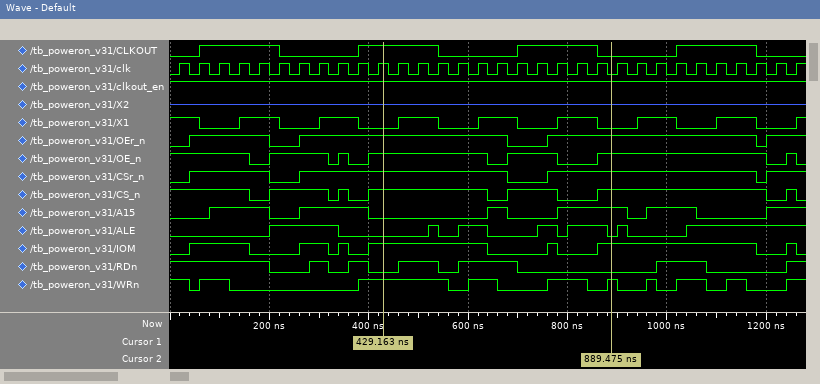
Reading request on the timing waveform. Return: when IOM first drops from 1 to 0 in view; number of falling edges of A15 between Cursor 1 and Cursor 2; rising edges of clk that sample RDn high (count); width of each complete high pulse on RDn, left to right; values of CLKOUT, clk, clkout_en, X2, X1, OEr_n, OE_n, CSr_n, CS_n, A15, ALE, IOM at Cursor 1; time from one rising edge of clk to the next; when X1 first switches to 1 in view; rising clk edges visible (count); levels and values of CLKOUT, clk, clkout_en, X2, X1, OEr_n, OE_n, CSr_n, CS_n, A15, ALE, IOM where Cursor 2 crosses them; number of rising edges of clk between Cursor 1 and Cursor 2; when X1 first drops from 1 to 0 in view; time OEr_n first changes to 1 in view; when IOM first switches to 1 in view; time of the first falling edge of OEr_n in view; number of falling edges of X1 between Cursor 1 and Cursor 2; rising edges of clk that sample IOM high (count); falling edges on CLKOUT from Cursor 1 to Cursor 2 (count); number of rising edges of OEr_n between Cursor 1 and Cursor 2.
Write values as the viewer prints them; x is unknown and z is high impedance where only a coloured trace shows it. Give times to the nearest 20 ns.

160 ns
1
15
40 ns, 40 ns, 80 ns, 120 ns, 100 ns
CLKOUT=1, clk=1, clkout_en=1, X2=z, X1=0, OEr_n=1, OE_n=1, CSr_n=1, CS_n=1, A15=0, ALE=0, IOM=1
40 ns
140 ns
32
CLKOUT=0, clk=0, clkout_en=1, X2=z, X1=0, OEr_n=1, OE_n=1, CSr_n=1, CS_n=1, A15=1, ALE=0, IOM=1
11
60 ns
40 ns
40 ns
200 ns
3
20
2
1
